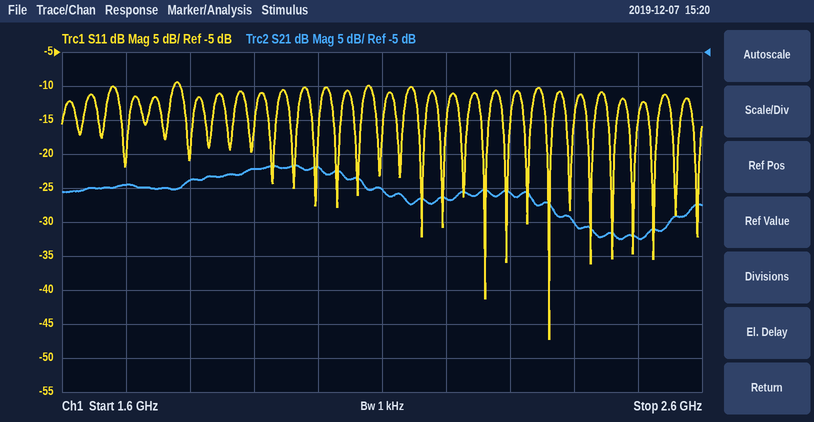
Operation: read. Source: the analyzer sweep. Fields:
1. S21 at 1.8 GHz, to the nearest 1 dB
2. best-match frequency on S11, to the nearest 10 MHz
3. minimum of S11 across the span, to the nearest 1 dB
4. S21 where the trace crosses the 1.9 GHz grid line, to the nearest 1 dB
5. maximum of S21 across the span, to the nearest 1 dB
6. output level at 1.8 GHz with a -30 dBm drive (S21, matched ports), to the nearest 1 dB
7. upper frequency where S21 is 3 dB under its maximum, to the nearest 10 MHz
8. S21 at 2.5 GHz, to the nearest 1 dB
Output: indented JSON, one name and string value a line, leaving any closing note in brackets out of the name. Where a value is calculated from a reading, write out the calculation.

{
  "S21 at 1.8 GHz, to the nearest 1 dB": "-24 dB",
  "best-match frequency on S11, to the nearest 10 MHz": "2.36 GHz",
  "minimum of S11 across the span, to the nearest 1 dB": "-47 dB",
  "S21 where the trace crosses the 1.9 GHz grid line, to the nearest 1 dB": "-22 dB",
  "maximum of S21 across the span, to the nearest 1 dB": "-22 dB",
  "output level at 1.8 GHz with a -30 dBm drive (S21, matched ports), to the nearest 1 dB": "-30 dBm + (-24 dB) = -54 dBm",
  "upper frequency where S21 is 3 dB under its maximum, to the nearest 10 MHz": "2.07 GHz",
  "S21 at 2.5 GHz, to the nearest 1 dB": "-32 dB"
}
